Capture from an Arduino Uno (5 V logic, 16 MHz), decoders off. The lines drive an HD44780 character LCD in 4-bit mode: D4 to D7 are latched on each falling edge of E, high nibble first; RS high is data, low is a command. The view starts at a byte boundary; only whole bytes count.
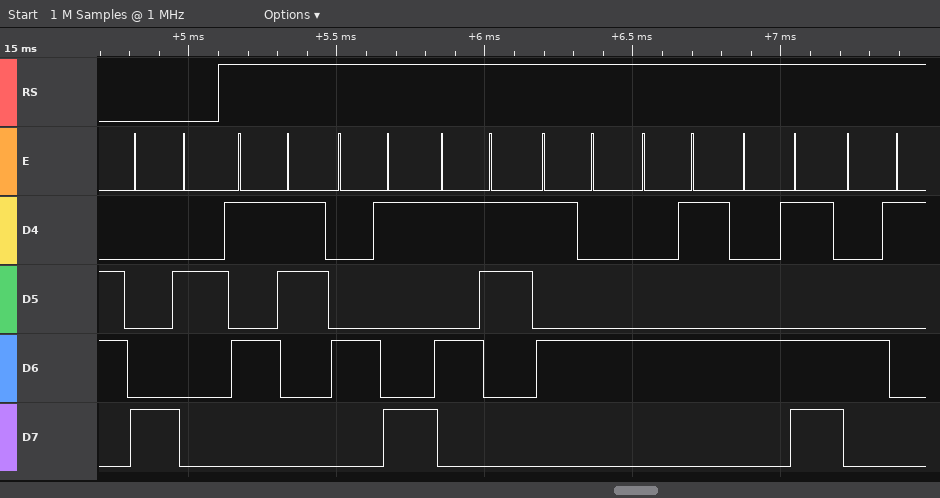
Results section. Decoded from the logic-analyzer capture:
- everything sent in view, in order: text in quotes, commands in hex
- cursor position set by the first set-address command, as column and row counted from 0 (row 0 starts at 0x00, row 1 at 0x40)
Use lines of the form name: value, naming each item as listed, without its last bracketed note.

everything sent in view, in order: text in quotes, commands in hex: 0x82 "SISTEMA"
cursor position set by the first set-address command, as column and row counted from 0: column 2, row 0
